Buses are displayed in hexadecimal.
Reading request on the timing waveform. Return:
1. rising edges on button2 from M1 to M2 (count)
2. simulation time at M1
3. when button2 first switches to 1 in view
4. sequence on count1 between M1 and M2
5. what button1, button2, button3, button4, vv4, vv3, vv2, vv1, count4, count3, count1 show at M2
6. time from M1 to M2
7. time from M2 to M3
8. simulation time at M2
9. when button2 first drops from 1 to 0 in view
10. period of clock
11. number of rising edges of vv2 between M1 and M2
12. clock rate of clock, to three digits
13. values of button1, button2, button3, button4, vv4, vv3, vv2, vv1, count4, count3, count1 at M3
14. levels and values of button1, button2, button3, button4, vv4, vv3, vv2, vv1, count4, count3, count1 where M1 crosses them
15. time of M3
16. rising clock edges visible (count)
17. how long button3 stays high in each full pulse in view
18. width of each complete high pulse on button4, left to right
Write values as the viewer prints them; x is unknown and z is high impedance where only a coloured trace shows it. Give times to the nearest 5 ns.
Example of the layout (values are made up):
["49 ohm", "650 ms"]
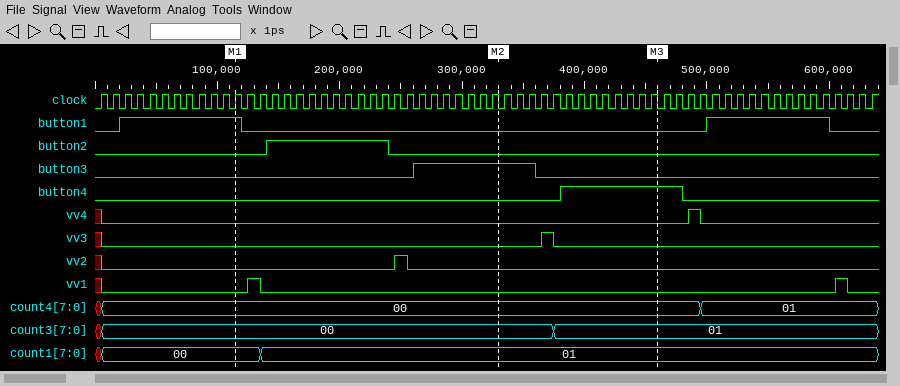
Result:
["1", "115 ns", "140 ns", "00, 01", "button1=0, button2=0, button3=1, button4=0, vv4=0, vv3=0, vv2=0, vv1=0, count4=00, count3=00, count1=01", "215 ns", "130 ns", "330 ns", "240 ns", "10 ns", "1", "100 MHz", "button1=0, button2=0, button3=0, button4=1, vv4=0, vv3=0, vv2=0, vv1=0, count4=00, count3=01, count1=01", "button1=1, button2=0, button3=0, button4=0, vv4=0, vv3=0, vv2=0, vv1=0, count4=00, count3=00, count1=00", "460 ns", "64", "100 ns", "100 ns"]
